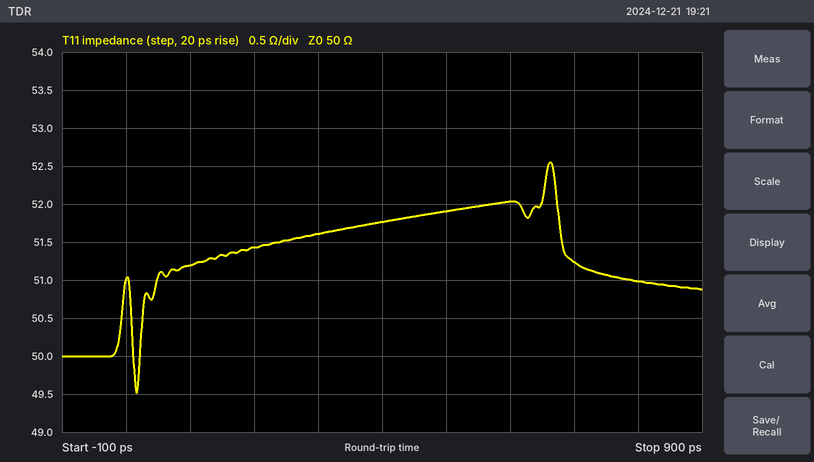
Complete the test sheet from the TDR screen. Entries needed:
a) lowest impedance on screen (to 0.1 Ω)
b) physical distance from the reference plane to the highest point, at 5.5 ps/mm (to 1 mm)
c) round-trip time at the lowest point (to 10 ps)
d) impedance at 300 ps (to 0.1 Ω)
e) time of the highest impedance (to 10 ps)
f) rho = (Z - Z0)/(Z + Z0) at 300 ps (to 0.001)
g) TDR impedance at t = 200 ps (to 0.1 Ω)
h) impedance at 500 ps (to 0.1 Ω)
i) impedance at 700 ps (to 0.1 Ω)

49.5 Ω
60 mm
20 ps
51.6 Ω
660 ps
+0.016
51.4 Ω
51.9 Ω
51.2 Ω
